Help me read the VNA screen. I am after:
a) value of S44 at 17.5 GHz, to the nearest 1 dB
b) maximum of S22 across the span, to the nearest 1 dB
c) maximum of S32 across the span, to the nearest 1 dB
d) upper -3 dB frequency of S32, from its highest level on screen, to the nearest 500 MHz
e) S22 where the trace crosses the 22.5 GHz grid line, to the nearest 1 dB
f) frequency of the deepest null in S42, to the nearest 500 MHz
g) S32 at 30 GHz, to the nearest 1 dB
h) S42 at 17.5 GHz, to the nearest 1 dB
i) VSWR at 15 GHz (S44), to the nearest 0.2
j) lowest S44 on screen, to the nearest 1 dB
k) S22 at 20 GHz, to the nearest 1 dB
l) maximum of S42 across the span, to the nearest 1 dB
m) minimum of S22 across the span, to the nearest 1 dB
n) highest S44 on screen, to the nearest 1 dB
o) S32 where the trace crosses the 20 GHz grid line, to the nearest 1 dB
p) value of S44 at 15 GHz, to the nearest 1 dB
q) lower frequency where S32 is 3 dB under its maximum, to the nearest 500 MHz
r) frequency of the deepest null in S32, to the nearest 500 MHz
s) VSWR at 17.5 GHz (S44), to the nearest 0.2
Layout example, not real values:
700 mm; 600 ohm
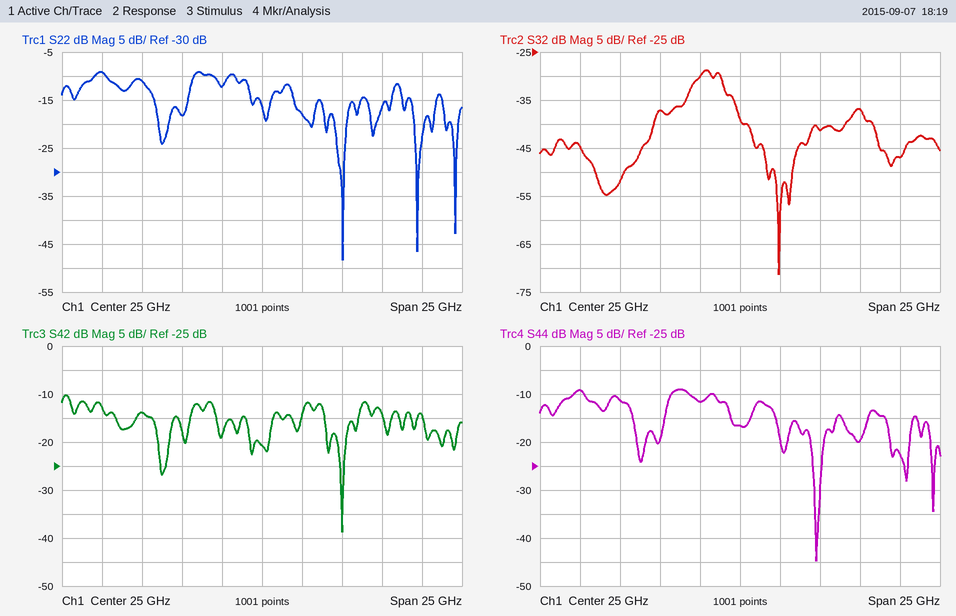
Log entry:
-11 dB; -9 dB; -29 dB; 24.0 GHz; -12 dB; 30.0 GHz; -41 dB; -14 dB; 2.0; -45 dB; -18 dB; -10 dB; -48 dB; -9 dB; -37 dB; -9 dB; 22.0 GHz; 27.5 GHz; 1.8
